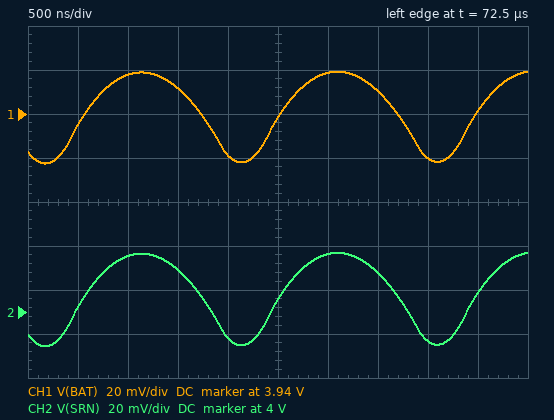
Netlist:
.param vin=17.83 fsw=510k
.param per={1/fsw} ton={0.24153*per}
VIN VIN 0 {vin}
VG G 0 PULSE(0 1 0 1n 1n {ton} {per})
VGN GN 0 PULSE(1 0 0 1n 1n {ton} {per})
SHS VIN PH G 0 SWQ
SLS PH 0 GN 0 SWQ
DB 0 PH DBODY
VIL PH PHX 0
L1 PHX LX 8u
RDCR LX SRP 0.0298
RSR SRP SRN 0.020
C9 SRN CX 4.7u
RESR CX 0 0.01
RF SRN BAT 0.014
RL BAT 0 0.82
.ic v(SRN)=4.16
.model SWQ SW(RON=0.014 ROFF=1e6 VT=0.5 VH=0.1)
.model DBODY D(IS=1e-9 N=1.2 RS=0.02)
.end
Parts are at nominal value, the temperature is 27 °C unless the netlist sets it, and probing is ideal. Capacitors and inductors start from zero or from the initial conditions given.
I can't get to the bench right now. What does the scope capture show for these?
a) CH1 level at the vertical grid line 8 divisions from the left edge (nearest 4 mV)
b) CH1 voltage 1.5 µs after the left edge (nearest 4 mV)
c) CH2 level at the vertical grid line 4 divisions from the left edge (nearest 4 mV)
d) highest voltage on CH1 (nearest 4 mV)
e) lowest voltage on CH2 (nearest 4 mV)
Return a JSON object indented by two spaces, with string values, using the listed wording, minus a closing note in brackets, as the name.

{
  "CH1 level at the vertical grid line 8 divisions from the left edge": "3.920 V",
  "CH1 voltage 1.5 µs after the left edge": "3.952 V",
  "CH2 level at the vertical grid line 4 divisions from the left edge": "3.988 V",
  "highest voltage on CH1": "3.960 V",
  "lowest voltage on CH2": "3.984 V"
}
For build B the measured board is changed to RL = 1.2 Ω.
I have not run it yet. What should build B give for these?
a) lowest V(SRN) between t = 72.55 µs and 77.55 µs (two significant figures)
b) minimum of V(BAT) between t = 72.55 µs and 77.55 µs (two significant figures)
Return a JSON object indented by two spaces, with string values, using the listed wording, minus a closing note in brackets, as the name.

{
  "lowest V(SRN) between t = 72.55 µs and 77.55 µs": "4.1 V",
  "minimum of V(BAT) between t = 72.55 µs and 77.55 µs": "4.0 V"
}
